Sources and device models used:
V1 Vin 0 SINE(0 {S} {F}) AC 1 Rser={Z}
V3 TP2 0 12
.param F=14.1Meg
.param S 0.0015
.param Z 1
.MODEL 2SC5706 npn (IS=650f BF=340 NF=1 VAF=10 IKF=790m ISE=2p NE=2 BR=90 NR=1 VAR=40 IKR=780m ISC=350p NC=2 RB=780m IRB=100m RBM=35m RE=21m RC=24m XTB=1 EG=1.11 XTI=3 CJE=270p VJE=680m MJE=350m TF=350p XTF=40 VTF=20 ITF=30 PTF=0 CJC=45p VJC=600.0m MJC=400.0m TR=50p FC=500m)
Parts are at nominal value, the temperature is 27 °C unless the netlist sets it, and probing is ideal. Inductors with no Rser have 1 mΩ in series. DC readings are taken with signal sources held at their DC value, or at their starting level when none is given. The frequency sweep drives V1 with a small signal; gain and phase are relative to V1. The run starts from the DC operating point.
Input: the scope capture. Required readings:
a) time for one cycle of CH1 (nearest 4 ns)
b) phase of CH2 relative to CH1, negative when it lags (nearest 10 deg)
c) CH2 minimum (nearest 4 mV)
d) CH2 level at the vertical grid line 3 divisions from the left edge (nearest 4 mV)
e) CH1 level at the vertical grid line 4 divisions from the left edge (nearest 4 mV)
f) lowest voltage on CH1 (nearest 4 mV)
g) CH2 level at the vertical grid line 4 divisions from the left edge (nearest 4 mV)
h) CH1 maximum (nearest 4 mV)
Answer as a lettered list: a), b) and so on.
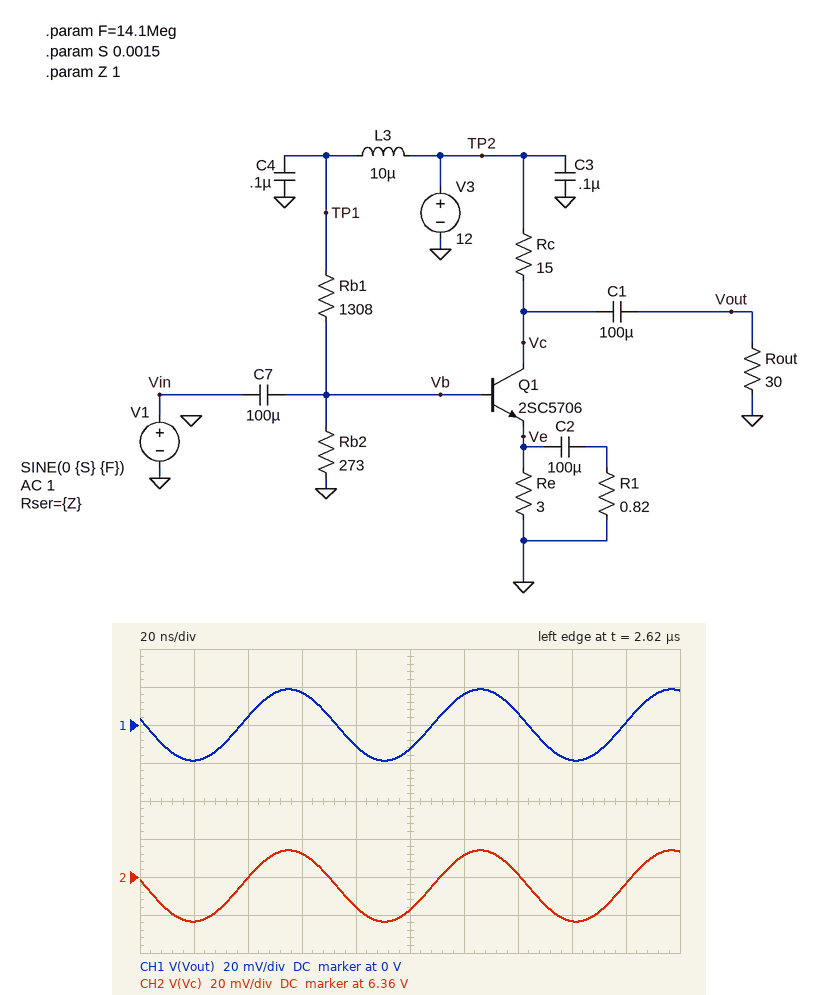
a) 72 ns
b) 0 deg
c) 6.336 V
d) 6.372 V
e) -12 mV
f) -20 mV
g) 6.344 V
h) 20 mV
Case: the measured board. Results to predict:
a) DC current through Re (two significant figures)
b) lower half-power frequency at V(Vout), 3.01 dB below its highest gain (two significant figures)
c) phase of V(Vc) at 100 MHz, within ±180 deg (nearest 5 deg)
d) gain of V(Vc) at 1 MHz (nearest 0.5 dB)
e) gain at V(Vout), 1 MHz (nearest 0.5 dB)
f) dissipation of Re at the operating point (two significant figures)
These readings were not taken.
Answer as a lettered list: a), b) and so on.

a) 380 mA
b) 1.6 kHz
c) 125 deg
d) 22.0 dB
e) 22.0 dB
f) 430 mW
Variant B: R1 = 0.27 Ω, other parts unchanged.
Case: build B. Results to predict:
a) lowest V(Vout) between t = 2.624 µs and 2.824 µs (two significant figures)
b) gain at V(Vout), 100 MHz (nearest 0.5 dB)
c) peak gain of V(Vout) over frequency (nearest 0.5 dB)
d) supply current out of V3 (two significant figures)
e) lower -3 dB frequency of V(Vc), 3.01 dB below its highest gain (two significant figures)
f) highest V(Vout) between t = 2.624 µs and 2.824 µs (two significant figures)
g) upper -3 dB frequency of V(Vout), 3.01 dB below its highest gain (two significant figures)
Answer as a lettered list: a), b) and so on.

a) -37 mV
b) 21.5 dB
c) 28.0 dB
d) 380 mA
e) 3.9 kHz
f) 37 mV
g) 51 MHz
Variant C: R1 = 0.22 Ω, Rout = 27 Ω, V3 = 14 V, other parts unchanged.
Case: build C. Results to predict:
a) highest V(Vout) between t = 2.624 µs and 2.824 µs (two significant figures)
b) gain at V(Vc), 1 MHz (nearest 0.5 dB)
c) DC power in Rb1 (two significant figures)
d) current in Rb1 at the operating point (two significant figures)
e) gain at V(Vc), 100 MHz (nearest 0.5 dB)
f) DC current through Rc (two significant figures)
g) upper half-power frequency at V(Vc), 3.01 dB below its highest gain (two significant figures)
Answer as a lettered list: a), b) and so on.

a) 42 mV
b) 29.5 dB
c) 110 mW
d) 9.1 mA
e) 21.5 dB
f) 470 mA
g) 46 MHz
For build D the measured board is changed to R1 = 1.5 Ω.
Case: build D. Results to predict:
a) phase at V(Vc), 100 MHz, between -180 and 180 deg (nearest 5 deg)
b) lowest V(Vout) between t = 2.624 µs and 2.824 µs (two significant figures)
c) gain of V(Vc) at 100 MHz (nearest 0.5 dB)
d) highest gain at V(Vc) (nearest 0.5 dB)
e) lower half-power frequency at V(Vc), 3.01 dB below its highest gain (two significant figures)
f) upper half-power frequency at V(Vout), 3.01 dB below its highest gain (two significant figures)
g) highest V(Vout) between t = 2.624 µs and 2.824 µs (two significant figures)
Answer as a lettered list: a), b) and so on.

a) 135 deg
b) -13 mV
c) 16.5 dB
d) 19.0 dB
e) 840 Hz
f) 120 MHz
g) 13 mV
